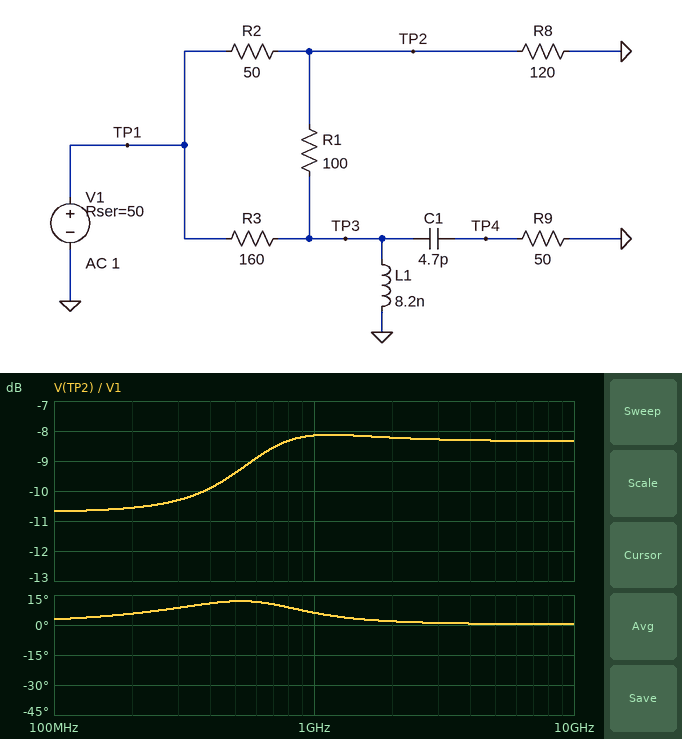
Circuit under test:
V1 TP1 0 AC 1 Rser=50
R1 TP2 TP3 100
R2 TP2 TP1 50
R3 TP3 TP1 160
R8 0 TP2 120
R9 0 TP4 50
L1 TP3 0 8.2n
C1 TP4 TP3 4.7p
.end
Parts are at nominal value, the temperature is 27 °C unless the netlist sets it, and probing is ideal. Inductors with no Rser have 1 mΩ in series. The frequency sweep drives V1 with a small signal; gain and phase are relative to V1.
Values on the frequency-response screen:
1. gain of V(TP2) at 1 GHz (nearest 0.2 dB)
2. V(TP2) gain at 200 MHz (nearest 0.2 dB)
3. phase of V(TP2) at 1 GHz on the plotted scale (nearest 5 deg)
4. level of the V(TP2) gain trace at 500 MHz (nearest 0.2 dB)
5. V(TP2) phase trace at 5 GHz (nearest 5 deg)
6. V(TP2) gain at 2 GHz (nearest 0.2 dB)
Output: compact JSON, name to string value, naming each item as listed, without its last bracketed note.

{"gain of V(TP2) at 1 GHz": "-8.2 dB", "V(TP2) gain at 200 MHz": "-10.6 dB", "phase of V(TP2) at 1 GHz on the plotted scale": "5 deg", "level of the V(TP2) gain trace at 500 MHz": "-9.4 dB", "V(TP2) phase trace at 5 GHz": "0 deg", "V(TP2) gain at 2 GHz": "-8.2 dB"}
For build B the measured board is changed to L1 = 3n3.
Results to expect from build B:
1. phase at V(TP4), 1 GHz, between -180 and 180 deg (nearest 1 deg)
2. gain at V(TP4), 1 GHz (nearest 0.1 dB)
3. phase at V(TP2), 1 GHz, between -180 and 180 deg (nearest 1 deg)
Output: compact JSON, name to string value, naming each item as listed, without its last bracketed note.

{"phase at V(TP4), 1 GHz, between -180 and 180 deg": "93 deg", "gain at V(TP4), 1 GHz": "-18.7 dB", "phase at V(TP2), 1 GHz, between -180 and 180 deg": "9 deg"}
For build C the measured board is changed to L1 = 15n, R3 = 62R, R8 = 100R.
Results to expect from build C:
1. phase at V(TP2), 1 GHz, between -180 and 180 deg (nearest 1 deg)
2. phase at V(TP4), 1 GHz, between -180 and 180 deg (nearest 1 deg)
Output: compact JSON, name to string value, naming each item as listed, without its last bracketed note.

{"phase at V(TP2), 1 GHz, between -180 and 180 deg": "1 deg", "phase at V(TP4), 1 GHz, between -180 and 180 deg": "37 deg"}
